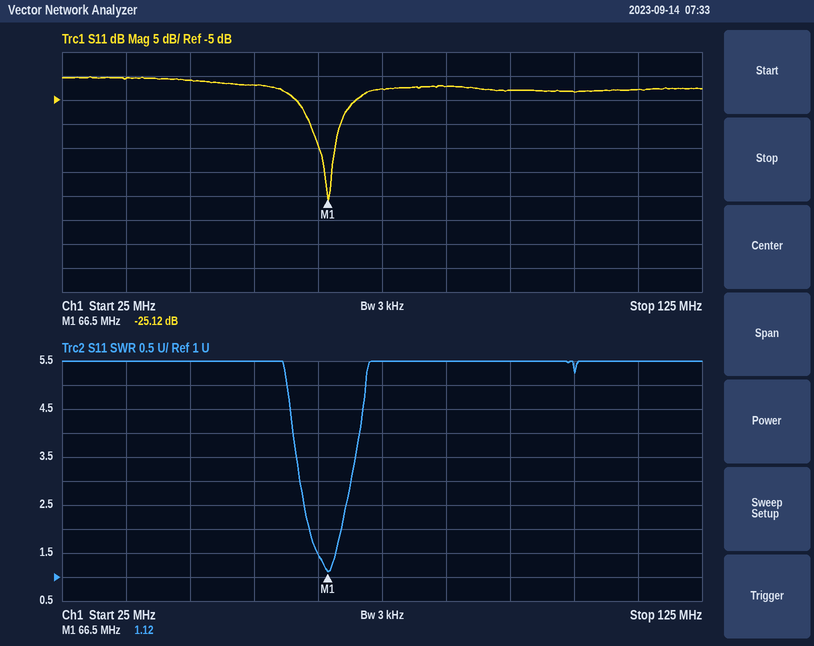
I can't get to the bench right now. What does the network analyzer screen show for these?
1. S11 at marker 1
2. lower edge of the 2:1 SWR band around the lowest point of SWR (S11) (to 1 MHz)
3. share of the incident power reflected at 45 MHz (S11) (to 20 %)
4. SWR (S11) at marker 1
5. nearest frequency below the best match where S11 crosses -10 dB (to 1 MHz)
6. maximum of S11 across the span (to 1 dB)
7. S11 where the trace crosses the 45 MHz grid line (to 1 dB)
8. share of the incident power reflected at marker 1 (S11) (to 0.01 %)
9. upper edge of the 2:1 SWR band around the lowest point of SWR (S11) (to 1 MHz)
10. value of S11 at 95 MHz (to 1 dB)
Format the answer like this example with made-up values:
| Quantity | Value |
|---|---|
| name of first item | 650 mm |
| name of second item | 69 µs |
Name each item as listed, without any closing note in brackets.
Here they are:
| Quantity | Value |
|---|---|
| S11 at marker 1 | -25.12 dB |
| lower edge of the 2:1 SWR band around the lowest point of SWR (S11) | 64 MHz |
| share of the incident power reflected at 45 MHz (S11) | 80 % |
| SWR (S11) at marker 1 | 1.12 |
| nearest frequency below the best match where S11 crosses -10 dB | 64 MHz |
| maximum of S11 across the span | 0 dB |
| S11 where the trace crosses the 45 MHz grid line | -1 dB |
| share of the incident power reflected at marker 1 (S11) | 0.31 % |
| upper edge of the 2:1 SWR band around the lowest point of SWR (S11) | 69 MHz |
| value of S11 at 95 MHz | -3 dB |
